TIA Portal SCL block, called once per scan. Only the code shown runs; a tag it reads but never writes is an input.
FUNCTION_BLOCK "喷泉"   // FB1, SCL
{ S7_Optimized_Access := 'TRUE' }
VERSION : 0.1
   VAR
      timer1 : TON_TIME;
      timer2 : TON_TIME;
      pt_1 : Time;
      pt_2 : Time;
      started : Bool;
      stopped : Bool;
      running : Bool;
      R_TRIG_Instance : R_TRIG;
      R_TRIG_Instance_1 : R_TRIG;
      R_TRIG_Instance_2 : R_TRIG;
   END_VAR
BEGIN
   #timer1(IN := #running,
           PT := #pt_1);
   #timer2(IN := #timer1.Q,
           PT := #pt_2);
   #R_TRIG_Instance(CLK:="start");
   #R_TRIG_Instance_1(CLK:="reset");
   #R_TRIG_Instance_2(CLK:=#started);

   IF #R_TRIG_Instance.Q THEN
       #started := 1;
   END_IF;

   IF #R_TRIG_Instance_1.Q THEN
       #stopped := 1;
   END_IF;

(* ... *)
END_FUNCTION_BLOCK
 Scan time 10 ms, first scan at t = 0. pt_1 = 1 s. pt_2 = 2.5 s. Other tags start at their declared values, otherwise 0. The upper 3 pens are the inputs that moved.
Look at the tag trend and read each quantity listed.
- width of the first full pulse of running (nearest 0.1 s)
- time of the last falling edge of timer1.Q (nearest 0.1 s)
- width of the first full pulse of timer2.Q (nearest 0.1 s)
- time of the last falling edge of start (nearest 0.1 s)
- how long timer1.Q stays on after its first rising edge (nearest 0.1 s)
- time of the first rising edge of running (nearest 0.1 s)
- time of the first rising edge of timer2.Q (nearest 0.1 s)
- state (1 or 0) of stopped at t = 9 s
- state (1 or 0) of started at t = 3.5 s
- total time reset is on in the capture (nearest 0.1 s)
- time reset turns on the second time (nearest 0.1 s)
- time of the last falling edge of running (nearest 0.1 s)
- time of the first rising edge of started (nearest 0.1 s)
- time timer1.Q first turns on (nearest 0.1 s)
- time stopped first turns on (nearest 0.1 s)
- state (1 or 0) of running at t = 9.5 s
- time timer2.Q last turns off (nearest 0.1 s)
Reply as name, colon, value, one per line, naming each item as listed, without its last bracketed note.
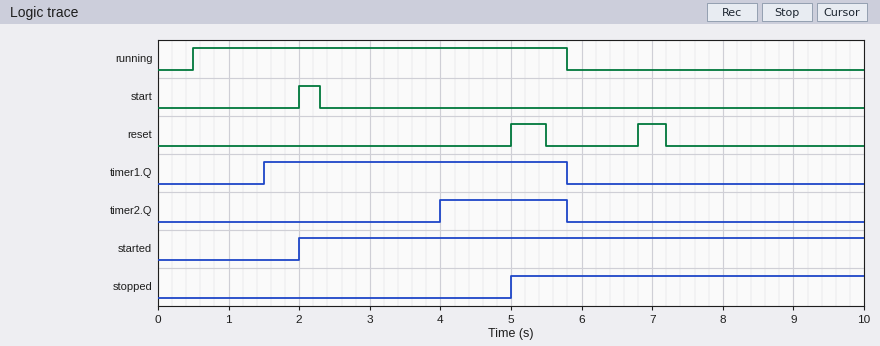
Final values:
width of the first full pulse of running: 5.3 s
time of the last falling edge of timer1.Q: 5.8 s
width of the first full pulse of timer2.Q: 1.8 s
time of the last falling edge of start: 2.3 s
how long timer1.Q stays on after its first rising edge: 4.3 s
time of the first rising edge of running: 0.5 s
time of the first rising edge of timer2.Q: 4.0 s
state (1 or 0) of stopped at t = 9 s: 1
state (1 or 0) of started at t = 3.5 s: 1
total time reset is on in the capture: 0.9 s
time reset turns on the second time: 6.8 s
time of the last falling edge of running: 5.8 s
time of the first rising edge of started: 2.0 s
time timer1.Q first turns on: 1.5 s
time stopped first turns on: 5.0 s
state (1 or 0) of running at t = 9.5 s: 0
time timer2.Q last turns off: 5.8 s
